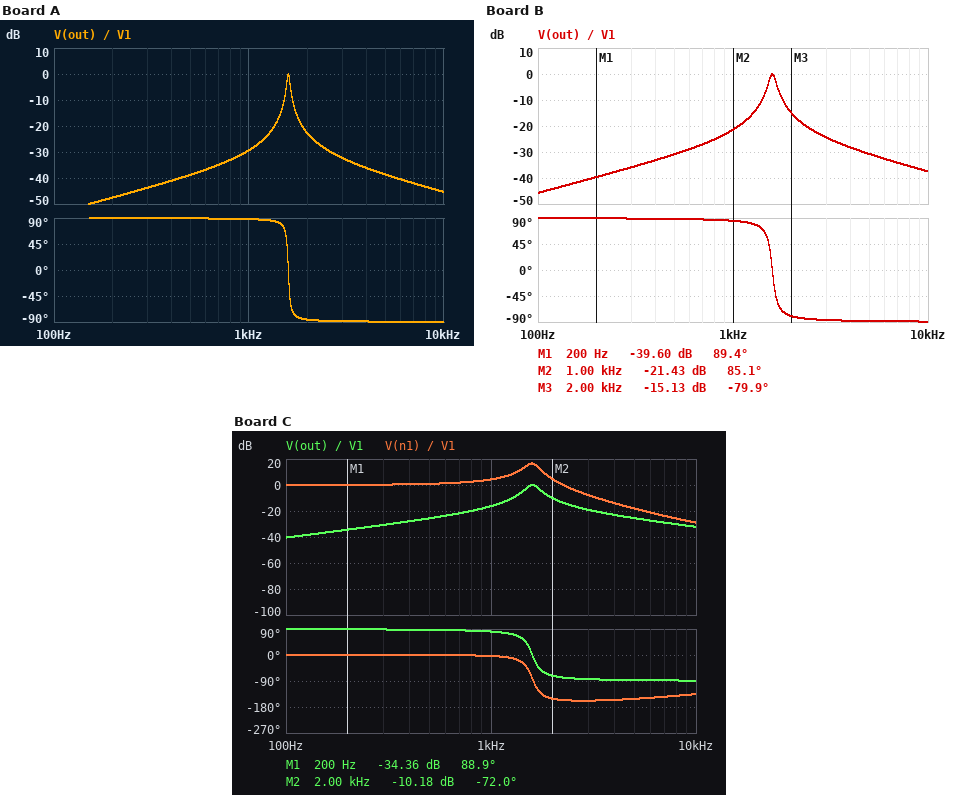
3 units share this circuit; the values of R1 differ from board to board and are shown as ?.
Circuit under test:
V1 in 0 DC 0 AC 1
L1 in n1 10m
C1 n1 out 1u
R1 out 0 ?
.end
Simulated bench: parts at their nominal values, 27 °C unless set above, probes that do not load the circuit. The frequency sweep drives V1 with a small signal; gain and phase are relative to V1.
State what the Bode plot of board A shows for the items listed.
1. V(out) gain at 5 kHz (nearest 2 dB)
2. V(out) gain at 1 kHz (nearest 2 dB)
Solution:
-38 dB
-30 dB
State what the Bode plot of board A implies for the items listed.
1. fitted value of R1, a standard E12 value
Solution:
3.3 Ω
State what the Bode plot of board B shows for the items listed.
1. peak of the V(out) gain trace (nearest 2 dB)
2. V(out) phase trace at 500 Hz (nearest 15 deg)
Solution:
0 dB
90 deg
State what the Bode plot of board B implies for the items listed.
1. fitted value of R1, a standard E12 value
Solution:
8.2 Ω
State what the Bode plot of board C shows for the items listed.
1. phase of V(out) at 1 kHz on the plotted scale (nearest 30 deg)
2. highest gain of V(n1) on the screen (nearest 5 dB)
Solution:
90 deg
15 dB
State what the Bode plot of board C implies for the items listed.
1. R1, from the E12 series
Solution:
15 Ω
